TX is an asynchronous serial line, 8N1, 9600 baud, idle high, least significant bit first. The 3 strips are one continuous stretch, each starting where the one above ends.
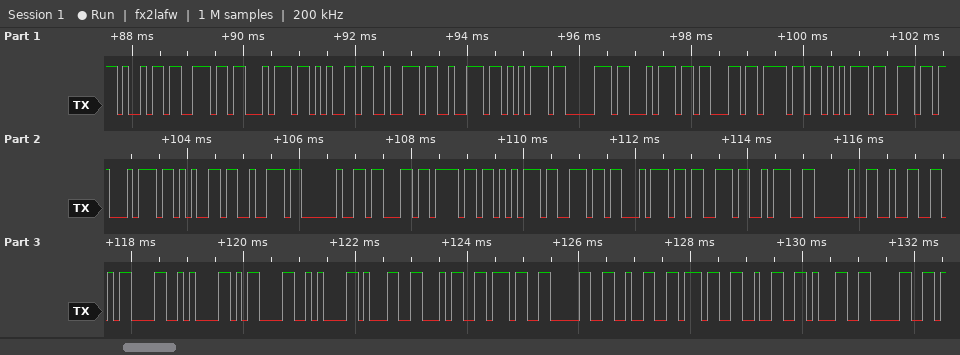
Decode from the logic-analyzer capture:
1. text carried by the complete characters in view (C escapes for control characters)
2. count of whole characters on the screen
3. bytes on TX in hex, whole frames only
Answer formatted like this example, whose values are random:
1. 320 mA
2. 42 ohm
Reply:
1. "interruptcounter counts: 2\r\n\r\n147027210"
2. 39
3. 69 6E 74 65 72 72 75 70 74 63 6F 75 6E 74 65 72 20 63 6F 75 6E 74 73 3A 20 32 0D 0A 0D 0A 31 34 37 30 32 37 32 31 30
